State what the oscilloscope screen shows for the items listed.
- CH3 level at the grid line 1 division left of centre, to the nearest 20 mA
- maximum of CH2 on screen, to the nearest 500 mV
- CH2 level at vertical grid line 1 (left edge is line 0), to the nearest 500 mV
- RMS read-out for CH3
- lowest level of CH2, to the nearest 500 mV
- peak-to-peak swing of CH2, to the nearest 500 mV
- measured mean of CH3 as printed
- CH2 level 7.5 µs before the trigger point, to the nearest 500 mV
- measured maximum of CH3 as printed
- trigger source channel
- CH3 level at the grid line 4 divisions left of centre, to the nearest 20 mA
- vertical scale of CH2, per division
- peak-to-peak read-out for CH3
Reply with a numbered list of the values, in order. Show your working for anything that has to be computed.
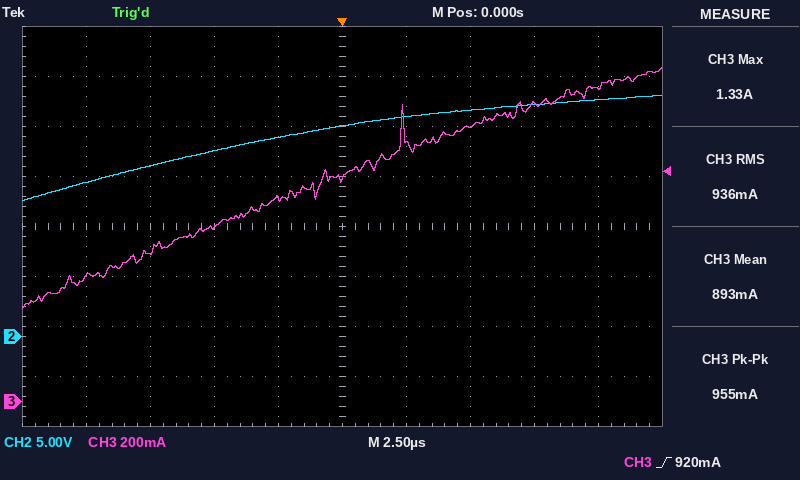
1. 820 mA
2. 24.0 V
3. 15.5 V
4. 936 mA
5. 13.5 V
6. 24.0 V − (13.5 V) = 10.5 V
7. 893 mA
8. 17.0 V
9. 1.33 A
10. CH3
11. 500 mA
12. 5 V
13. 955 mA
